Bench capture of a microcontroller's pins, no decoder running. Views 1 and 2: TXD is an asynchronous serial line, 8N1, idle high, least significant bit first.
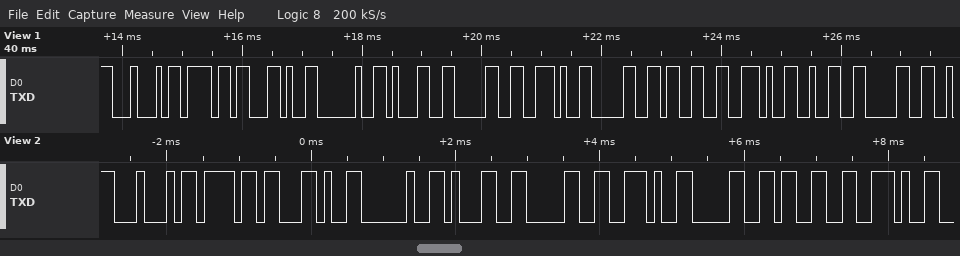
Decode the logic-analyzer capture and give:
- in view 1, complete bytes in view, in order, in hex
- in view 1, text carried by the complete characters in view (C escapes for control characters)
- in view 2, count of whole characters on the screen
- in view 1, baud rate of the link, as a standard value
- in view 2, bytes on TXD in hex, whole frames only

44 6F 2C 20 31 30 2E 30 33 2E 32 30
"Do, 10.03.20"
10
9600 baud
0x44 0x6F 0x2C 0x20 0x31 0x30 0x2E 0x30 0x33 0x2E
